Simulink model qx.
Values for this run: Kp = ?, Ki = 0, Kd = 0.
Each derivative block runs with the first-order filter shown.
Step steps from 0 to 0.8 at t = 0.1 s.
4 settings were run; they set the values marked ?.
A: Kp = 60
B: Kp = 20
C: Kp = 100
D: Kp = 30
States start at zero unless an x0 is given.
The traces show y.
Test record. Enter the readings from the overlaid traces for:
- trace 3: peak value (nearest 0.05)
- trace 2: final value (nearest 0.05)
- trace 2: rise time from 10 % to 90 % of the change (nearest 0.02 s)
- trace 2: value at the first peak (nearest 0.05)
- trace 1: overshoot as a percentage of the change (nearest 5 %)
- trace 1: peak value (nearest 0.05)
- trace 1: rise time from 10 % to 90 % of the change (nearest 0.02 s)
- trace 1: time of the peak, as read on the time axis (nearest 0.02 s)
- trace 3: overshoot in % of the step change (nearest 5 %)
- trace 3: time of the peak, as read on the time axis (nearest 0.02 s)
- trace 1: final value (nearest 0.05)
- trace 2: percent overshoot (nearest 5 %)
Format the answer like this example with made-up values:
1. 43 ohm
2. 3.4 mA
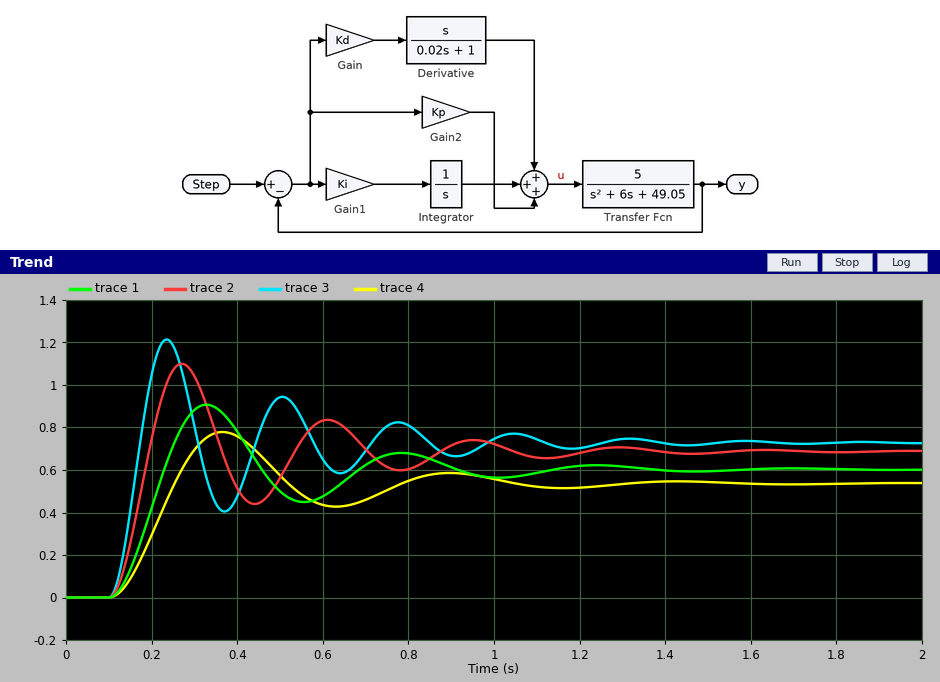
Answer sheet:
1. 1.20
2. 0.70
3. 0.06 s
4. 1.10
5. 50 %
6. 0.90
7. 0.08 s
8. 0.32 s
9. 65 %
10. 0.24 s
11. 0.60
12. 60 %
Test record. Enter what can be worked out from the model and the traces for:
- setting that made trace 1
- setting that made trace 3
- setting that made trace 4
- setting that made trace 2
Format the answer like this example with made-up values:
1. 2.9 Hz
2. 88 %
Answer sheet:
1. D
2. C
3. B
4. A
